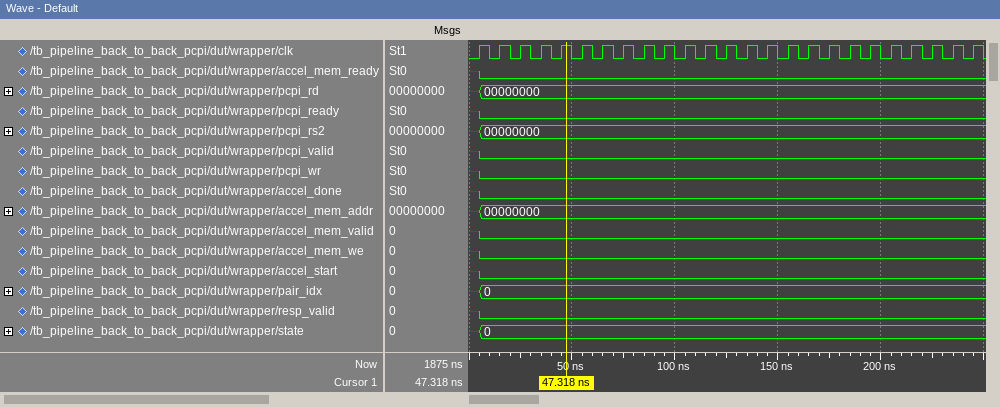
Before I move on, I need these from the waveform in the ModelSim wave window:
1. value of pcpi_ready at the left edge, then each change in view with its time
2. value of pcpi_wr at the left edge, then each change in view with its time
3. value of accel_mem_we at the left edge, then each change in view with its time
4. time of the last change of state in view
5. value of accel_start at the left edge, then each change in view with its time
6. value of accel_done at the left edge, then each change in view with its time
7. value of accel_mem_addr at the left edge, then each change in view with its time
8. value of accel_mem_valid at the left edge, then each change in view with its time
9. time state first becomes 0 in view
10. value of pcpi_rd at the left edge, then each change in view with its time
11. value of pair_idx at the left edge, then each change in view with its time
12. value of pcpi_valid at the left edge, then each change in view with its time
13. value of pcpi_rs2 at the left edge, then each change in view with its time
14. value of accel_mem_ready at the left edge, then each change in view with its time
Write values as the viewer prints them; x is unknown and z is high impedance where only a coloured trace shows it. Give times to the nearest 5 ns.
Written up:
x, 0 at 5 ns
x, 0 at 5 ns
x, 0 at 5 ns
5 ns
x, 0 at 5 ns
x, 0 at 5 ns
x, 00000000 at 5 ns
x, 0 at 5 ns
5 ns
x, 00000000 at 5 ns
x, 0 at 5 ns
x, 0 at 5 ns
x, 00000000 at 5 ns
x, 0 at 5 ns
